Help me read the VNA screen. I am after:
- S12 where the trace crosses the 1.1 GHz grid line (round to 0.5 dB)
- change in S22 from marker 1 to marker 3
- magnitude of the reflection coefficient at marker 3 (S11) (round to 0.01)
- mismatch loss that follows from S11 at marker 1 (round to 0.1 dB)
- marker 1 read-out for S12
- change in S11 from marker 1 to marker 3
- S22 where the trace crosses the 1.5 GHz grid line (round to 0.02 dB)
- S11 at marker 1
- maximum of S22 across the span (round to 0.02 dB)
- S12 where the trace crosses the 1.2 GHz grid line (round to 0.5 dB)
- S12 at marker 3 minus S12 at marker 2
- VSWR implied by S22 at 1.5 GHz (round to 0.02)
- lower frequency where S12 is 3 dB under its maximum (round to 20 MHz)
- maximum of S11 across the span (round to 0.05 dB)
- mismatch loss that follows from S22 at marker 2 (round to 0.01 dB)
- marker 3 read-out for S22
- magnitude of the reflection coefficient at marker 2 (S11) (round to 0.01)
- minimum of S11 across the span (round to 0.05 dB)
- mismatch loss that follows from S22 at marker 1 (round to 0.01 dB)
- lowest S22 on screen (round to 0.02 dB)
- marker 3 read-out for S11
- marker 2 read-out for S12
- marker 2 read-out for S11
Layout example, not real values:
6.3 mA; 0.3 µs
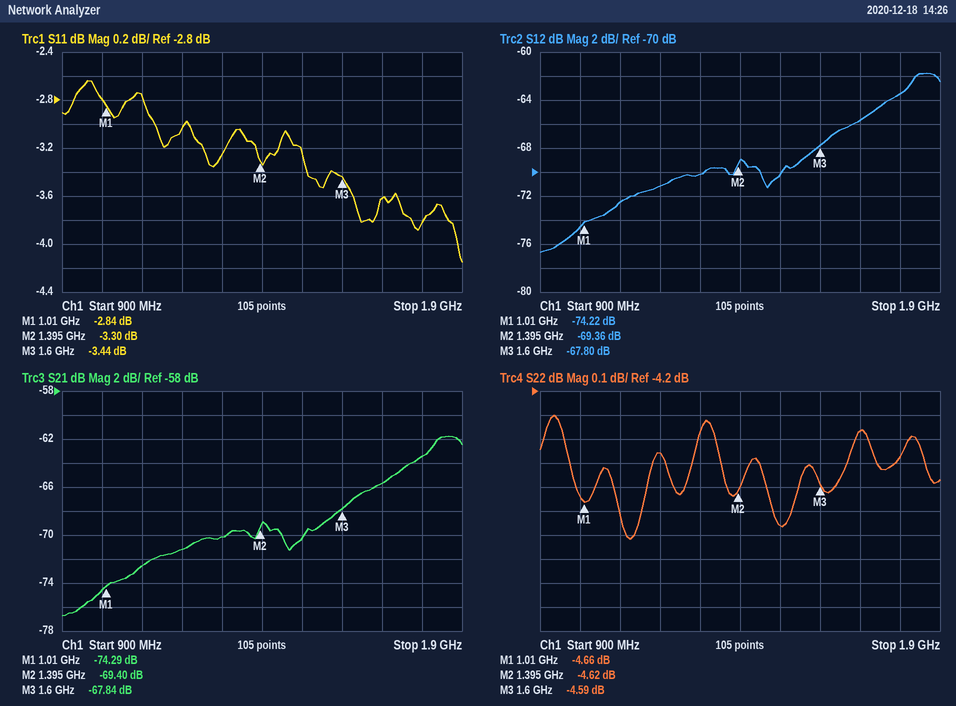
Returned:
-72.5 dB; 0.07 dB; 0.67; 3.2 dB; -74.22 dB; -0.60 dB; -4.76 dB; -2.84 dB; -4.30 dB; -71.0 dB; 1.56 dB; 3.74; 1.74 GHz; -2.65 dB; 1.84 dB; -4.59 dB; 0.68; -4.15 dB; 1.82 dB; -4.82 dB; -3.44 dB; -69.36 dB; -3.30 dB
